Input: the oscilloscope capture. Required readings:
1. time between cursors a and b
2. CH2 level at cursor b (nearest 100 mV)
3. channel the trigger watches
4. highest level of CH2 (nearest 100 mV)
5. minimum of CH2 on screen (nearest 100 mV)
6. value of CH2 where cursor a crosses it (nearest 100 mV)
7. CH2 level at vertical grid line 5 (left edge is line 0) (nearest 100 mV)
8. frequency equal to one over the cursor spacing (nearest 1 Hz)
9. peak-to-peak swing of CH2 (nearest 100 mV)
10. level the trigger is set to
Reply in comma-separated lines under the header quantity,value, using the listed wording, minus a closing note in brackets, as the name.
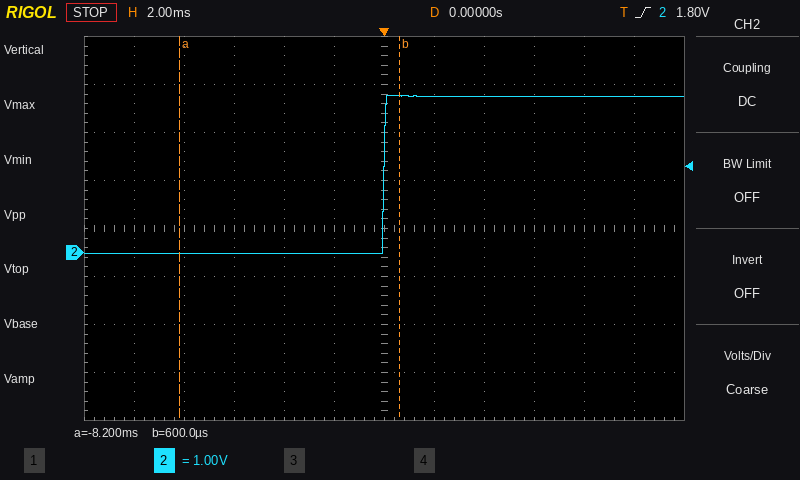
quantity,value
time between cursors a and b,8.8 ms
CH2 level at cursor b,3.3 V
channel the trigger watches,CH2
highest level of CH2,3.3 V
minimum of CH2 on screen,0.0 V
value of CH2 where cursor a crosses it,0.0 V
CH2 level at vertical grid line 5 (left edge is line 0),0.0 V
frequency equal to one over the cursor spacing,114 Hz
peak-to-peak swing of CH2,3.3 V
level the trigger is set to,1.80 V
